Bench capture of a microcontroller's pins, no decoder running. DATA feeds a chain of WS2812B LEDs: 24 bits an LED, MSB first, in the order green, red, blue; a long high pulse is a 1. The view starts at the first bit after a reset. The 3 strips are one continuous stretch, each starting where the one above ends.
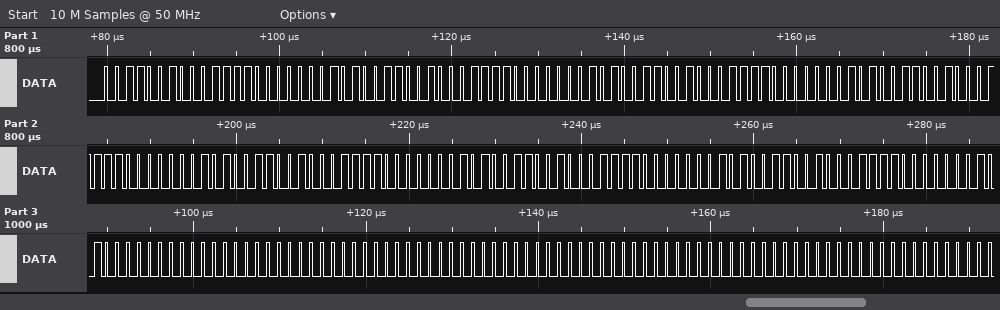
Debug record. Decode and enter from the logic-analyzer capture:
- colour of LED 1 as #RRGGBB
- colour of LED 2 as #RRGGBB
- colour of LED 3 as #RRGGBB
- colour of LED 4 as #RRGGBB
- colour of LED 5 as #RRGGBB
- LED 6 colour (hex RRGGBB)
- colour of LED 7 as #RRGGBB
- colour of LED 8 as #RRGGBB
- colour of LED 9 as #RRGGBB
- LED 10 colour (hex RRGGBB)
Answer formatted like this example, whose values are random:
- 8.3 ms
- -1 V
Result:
- #3C3205
- #3C3205
- #3C3205
- #3C3205
- #3C3205
- #3C3205
- #3C3205
- #000000
- #000000
- #000000
